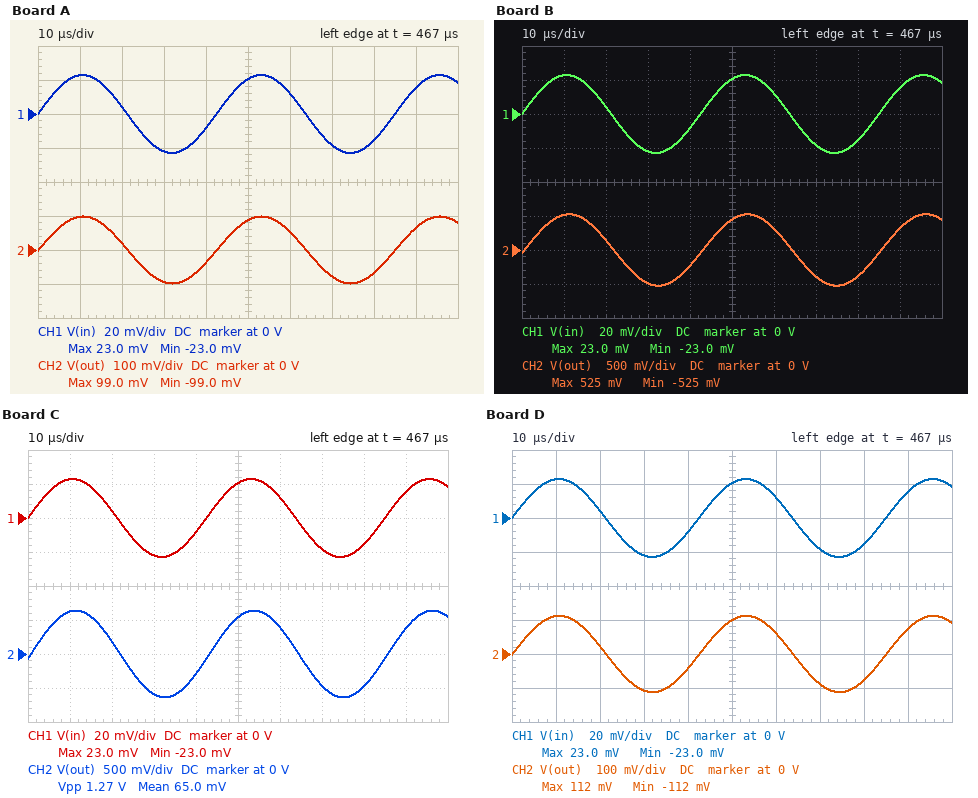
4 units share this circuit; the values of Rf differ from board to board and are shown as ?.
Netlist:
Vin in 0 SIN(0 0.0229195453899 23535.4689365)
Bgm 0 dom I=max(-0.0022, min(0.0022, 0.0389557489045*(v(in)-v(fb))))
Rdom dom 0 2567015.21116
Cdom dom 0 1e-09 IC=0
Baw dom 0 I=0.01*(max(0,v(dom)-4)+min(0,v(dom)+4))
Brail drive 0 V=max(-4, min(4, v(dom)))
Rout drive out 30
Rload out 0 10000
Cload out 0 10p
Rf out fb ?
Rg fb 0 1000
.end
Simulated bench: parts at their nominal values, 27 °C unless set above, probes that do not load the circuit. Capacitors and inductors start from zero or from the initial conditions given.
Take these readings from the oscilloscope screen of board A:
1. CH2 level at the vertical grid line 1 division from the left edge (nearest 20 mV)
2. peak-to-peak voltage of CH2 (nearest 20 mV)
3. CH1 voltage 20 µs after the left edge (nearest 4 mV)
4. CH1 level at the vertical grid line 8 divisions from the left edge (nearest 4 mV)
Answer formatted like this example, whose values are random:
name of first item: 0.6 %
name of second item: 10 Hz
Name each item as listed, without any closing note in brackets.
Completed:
CH2 level at the vertical grid line 1 division from the left edge: 100 mV
peak-to-peak voltage of CH2: 200 mV
CH1 voltage 20 µs after the left edge: 4 mV
CH1 level at the vertical grid line 8 divisions from the left edge: -16 mV
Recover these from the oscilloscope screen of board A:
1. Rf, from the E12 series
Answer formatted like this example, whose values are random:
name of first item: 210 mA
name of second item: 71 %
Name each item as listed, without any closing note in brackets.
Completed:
Rf, from the E12 series: 3.3 kΩ
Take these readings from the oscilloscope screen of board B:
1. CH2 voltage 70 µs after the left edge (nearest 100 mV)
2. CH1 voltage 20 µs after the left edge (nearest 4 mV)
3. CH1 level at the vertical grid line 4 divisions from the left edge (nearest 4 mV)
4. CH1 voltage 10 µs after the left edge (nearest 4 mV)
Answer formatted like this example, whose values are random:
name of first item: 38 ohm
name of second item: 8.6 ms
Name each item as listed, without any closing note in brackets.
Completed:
CH2 voltage 70 µs after the left edge: -400 mV
CH1 voltage 20 µs after the left edge: 4 mV
CH1 level at the vertical grid line 4 divisions from the left edge: -8 mV
CH1 voltage 10 µs after the left edge: 24 mV
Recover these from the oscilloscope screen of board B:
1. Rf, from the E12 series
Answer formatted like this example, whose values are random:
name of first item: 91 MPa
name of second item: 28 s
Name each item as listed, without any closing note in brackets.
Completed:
Rf, from the E12 series: 22 kΩ
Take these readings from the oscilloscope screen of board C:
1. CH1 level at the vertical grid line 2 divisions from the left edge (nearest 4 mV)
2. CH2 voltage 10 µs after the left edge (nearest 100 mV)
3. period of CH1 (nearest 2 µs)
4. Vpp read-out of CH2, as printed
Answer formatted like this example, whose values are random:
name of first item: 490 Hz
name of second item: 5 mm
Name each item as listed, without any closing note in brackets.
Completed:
CH1 level at the vertical grid line 2 divisions from the left edge: 4 mV
CH2 voltage 10 µs after the left edge: 600 mV
period of CH1: 42 µs
Vpp read-out of CH2, as printed: 1.27 V
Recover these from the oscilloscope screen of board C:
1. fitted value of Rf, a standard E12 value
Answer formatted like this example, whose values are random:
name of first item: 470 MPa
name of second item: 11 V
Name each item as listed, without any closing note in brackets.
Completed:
fitted value of Rf, a standard E12 value: 27 kΩ
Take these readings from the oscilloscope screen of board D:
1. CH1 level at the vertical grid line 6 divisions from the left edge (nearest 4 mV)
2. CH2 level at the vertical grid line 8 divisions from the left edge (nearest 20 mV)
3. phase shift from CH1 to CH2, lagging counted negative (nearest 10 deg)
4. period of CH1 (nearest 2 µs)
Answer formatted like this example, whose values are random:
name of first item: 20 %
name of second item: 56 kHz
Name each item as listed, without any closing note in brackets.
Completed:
CH1 level at the vertical grid line 6 divisions from the left edge: 12 mV
CH2 level at the vertical grid line 8 divisions from the left edge: -80 mV
phase shift from CH1 to CH2, lagging counted negative: 0 deg
period of CH1: 42 µs
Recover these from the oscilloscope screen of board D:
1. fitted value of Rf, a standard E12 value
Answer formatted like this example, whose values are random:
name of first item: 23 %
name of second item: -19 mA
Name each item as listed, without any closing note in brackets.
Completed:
fitted value of Rf, a standard E12 value: 3.9 kΩ
